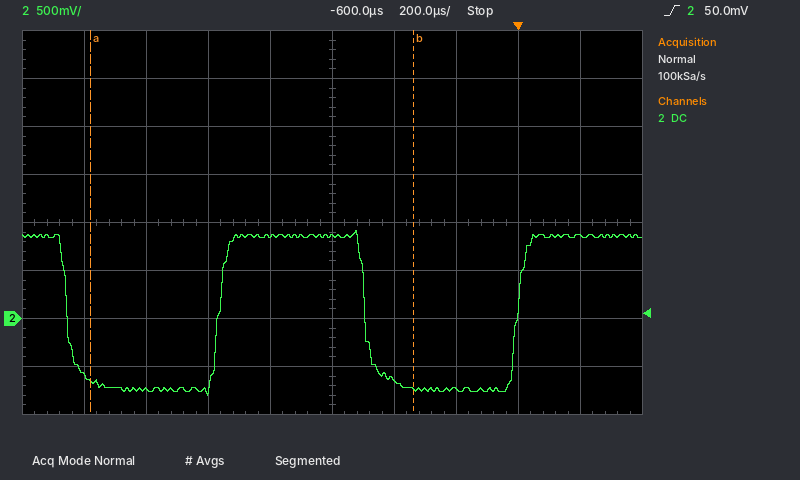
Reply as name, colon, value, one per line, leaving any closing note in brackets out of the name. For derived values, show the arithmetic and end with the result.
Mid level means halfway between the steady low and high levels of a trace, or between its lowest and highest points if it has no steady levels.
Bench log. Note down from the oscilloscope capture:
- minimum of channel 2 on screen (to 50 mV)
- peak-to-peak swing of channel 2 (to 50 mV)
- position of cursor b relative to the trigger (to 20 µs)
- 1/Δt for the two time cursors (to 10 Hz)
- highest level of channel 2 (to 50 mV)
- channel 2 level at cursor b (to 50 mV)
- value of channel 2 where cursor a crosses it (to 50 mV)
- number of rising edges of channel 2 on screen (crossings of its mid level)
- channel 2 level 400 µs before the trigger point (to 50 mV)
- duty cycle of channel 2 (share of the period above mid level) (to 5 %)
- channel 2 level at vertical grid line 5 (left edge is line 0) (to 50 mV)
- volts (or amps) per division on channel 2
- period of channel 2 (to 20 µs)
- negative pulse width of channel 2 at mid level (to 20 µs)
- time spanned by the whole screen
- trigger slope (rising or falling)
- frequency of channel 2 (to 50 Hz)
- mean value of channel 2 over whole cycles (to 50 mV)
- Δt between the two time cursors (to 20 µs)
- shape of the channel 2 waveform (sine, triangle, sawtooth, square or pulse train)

minimum of channel 2 on screen: -800 mV
peak-to-peak swing of channel 2: 900 mV − (-800 mV) = 1.70 V
position of cursor b relative to the trigger: -340 µs
1/Δt for the two time cursors: 1 / 1.04 ms ≈ 960 Hz
highest level of channel 2: 900 mV
channel 2 level at cursor b: -750 mV
value of channel 2 where cursor a crosses it: -650 mV
number of rising edges of channel 2 on screen: 2
channel 2 level 400 µs before the trigger point: -650 mV
duty cycle of channel 2 (share of the period above mid level): 50 %
channel 2 level at vertical grid line 5 (left edge is line 0): 850 mV
volts (or amps) per division on channel 2: 500 mV
period of channel 2: 960 µs
negative pulse width of channel 2 at mid level: 500 µs
time spanned by the whole screen: 2 ms
trigger slope: rising
frequency of channel 2: 1 / 960 µs ≈ 1.04 kHz, so 1.05 kHz to the nearest 50 Hz
mean value of channel 2 over whole cycles: -800 mV + 0.5 × (900 mV − (-800 mV)) ≈ 50 mV
Δt between the two time cursors: 1.04 ms
shape of the channel 2 waveform: square
